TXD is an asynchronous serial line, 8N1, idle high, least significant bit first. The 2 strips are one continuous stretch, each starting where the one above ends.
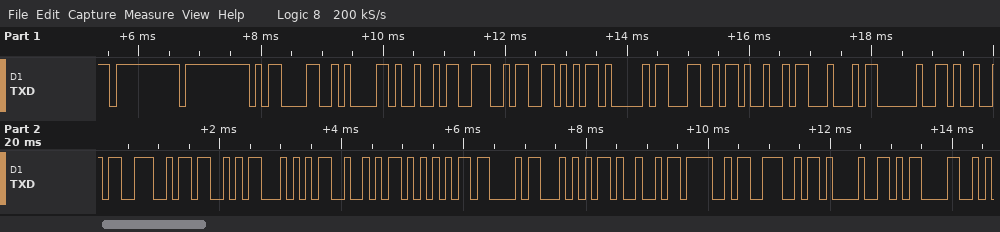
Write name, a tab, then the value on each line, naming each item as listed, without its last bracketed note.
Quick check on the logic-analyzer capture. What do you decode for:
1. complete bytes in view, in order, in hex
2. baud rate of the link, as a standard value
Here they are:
complete bytes in view, in order, in hex	0xFF 0xFF 0x0D 0x0A 0x49 0x4E 0x56 0x41 0x4C 0x49 0x44 0x20 0x49 0x4E 0x53 0x54 0x52 0x55 0x43 0x54 0x49 0x4F 0x4E 0x21 0x0D
baud rate of the link, as a standard value	9600 baud
